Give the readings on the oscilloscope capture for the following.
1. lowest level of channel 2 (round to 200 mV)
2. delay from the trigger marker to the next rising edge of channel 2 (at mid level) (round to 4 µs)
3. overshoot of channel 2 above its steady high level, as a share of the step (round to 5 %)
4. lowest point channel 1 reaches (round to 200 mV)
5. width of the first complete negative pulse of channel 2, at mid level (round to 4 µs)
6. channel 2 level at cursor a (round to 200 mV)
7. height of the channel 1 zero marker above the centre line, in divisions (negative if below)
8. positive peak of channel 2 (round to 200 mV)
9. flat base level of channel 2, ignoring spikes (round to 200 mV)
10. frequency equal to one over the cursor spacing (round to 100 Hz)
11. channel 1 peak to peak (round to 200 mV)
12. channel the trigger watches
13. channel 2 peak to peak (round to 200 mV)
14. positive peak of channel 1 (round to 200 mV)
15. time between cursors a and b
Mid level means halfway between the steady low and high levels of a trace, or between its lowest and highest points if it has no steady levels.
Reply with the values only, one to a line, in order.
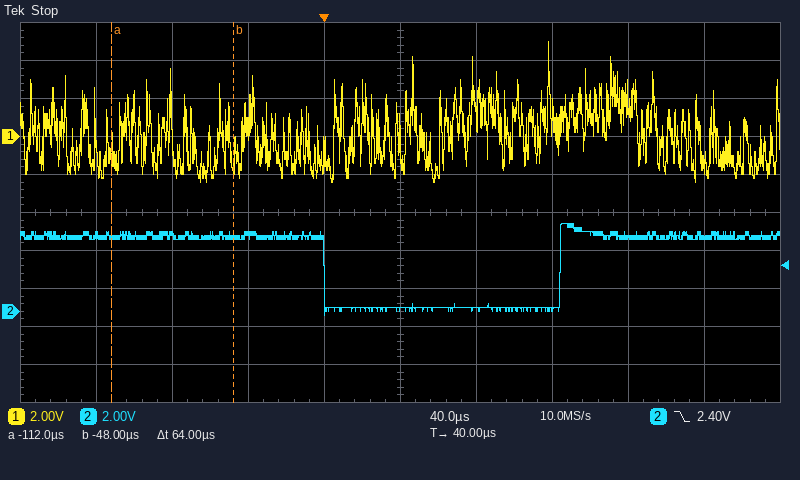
-200 mV
124 µs
20 %
-2.4 V
124 µs
4.0 V
+2.0 div
4.6 V
200 mV
15.6 kHz
7.4 V
channel 2
4.8 V
5.0 V
64 µs
